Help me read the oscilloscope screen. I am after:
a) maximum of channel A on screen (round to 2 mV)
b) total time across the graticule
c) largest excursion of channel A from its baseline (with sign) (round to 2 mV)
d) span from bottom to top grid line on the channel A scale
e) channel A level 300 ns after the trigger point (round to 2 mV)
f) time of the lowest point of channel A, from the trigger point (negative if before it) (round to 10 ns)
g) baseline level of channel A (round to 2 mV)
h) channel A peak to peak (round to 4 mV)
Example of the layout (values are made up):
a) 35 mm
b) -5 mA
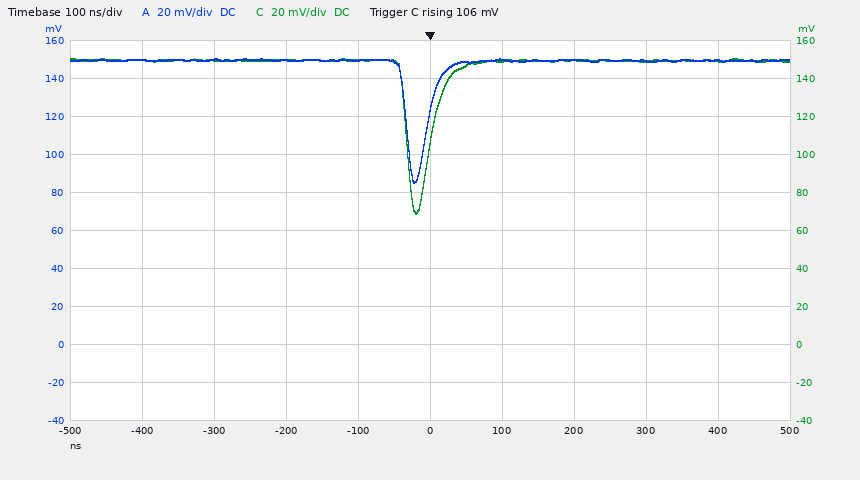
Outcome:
a) 150 mV
b) 1 µs
c) -64 mV
d) 200 mV
e) 150 mV
f) -20 ns
g) 150 mV
h) 64 mV
